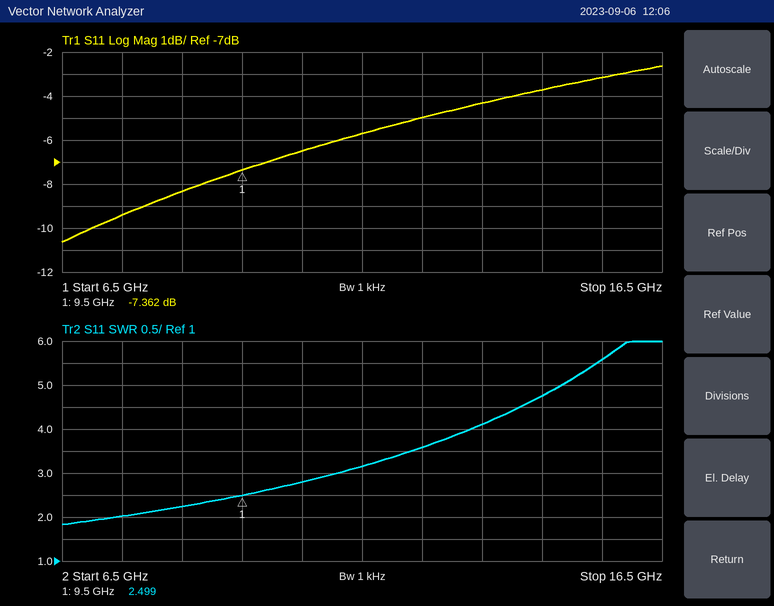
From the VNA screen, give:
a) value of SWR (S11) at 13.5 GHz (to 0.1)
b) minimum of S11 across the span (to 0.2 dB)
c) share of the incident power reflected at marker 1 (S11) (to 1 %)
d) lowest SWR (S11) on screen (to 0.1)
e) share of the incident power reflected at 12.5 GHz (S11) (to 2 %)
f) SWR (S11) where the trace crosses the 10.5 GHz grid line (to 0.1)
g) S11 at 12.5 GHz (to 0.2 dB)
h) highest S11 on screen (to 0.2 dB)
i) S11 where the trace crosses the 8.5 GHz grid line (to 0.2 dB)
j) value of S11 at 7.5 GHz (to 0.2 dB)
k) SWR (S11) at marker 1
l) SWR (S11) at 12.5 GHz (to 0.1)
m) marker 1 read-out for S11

4.1
-10.6 dB
18 %
1.8
32 %
2.8
-5.0 dB
-2.6 dB
-8.4 dB
-9.4 dB
2.499
3.6
-7.362 dB
